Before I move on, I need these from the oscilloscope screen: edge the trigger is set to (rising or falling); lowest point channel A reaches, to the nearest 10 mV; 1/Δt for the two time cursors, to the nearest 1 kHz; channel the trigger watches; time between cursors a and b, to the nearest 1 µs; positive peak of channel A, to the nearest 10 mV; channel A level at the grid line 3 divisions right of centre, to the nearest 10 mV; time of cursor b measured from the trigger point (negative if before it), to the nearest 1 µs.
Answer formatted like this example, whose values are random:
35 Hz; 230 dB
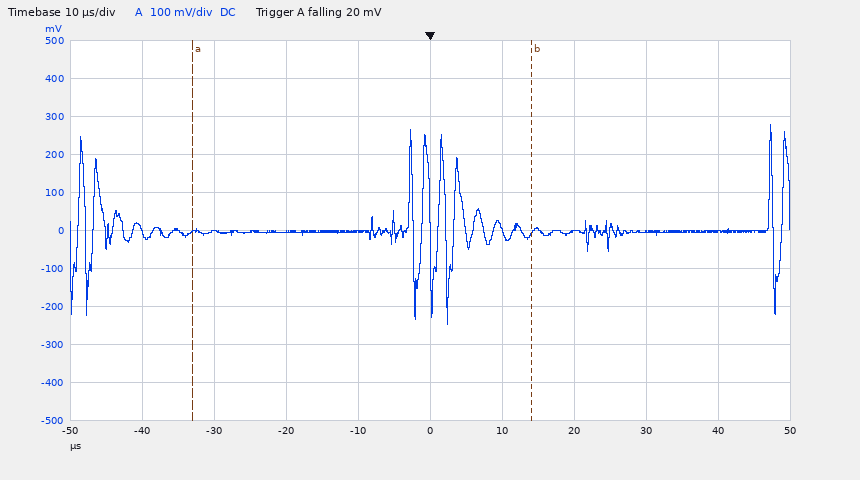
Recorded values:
falling; -250 mV; 21 kHz; channel A; 47 µs; 280 mV; 0 mV; +14 µs
